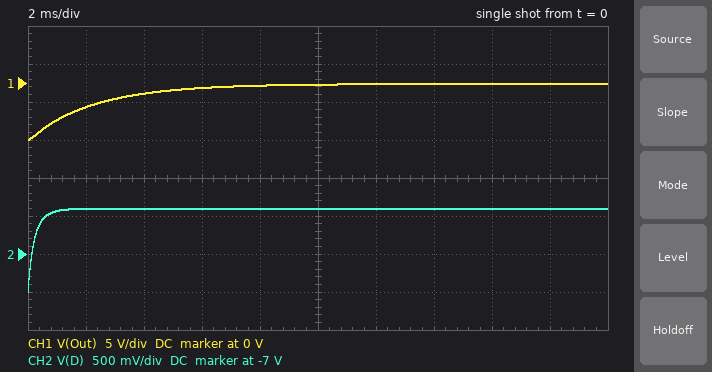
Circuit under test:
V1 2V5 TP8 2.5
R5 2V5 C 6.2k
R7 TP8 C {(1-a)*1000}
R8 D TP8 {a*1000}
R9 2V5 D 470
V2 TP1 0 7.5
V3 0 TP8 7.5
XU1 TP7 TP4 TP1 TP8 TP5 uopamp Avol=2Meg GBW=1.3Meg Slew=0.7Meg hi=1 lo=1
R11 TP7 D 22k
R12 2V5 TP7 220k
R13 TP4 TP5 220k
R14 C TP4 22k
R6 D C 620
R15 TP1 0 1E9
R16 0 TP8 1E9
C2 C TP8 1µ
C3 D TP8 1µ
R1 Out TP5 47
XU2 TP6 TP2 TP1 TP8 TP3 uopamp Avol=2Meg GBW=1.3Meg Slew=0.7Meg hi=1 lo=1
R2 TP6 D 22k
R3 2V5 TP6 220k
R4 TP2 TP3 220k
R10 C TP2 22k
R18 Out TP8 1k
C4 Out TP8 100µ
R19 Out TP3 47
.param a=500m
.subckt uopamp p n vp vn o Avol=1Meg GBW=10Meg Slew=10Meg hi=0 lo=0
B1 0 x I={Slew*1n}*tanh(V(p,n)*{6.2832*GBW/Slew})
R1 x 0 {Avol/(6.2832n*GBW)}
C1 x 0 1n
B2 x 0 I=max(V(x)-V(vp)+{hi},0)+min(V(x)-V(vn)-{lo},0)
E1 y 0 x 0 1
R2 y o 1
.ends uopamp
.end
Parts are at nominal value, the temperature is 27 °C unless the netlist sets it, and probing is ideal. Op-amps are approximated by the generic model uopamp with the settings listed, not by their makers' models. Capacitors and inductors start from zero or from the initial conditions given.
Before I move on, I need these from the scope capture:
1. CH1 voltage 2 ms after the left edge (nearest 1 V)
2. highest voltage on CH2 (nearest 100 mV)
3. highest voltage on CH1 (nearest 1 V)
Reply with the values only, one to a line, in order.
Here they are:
-3 V
-6.4 V
0 V
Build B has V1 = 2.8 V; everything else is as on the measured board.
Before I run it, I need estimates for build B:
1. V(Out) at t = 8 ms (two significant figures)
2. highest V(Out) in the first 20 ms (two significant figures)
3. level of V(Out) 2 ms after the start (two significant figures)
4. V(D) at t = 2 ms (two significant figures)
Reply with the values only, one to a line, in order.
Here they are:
510 mV
760 mV
-2.7 V
-6.3 V
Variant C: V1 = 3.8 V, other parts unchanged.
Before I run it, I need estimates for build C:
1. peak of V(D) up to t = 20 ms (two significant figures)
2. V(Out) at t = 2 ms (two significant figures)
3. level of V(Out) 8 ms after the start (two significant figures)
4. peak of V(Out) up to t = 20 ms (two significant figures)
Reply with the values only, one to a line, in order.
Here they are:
-5.8 V
-940 mV
3.4 V
3.7 V
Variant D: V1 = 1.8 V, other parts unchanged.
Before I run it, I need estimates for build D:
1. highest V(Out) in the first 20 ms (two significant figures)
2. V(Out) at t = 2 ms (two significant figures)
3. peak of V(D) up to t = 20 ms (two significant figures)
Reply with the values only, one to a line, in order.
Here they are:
-2.2 V
-4.4 V
-6.7 V
